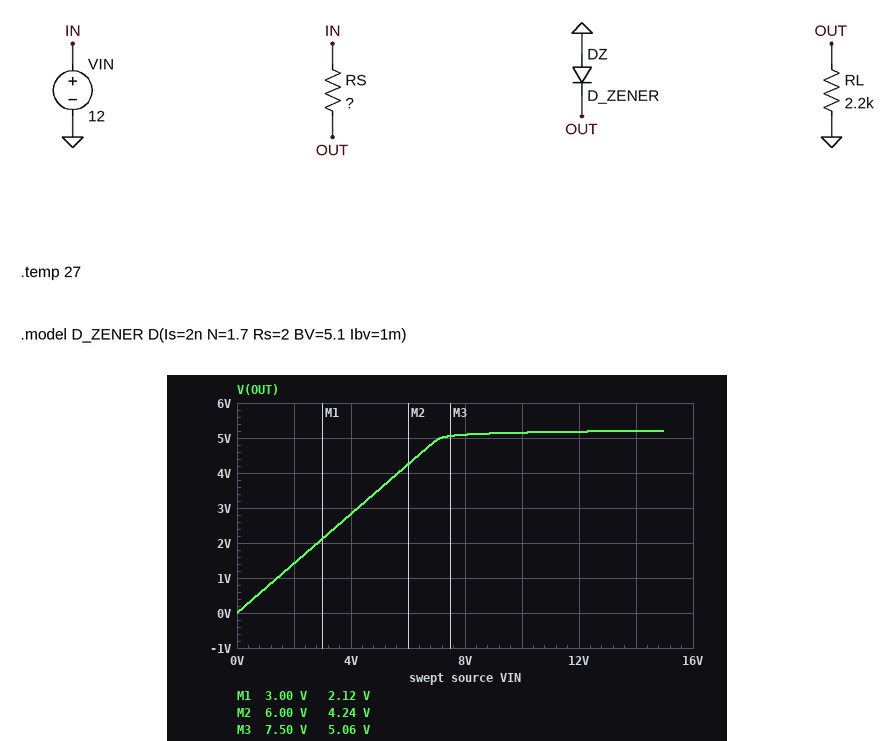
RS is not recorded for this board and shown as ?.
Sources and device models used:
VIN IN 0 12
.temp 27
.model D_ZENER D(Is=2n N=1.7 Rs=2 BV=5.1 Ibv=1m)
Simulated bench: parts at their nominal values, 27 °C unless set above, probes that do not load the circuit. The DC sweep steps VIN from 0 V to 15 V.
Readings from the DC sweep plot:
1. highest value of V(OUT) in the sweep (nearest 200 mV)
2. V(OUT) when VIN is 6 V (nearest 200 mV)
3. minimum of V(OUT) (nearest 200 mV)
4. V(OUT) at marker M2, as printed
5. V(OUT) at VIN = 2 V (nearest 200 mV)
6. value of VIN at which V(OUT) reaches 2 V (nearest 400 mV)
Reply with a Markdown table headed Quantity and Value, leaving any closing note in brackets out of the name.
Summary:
| Quantity | Value |
|---|---|
| highest value of V(OUT) in the sweep | 5.2 V |
| V(OUT) when VIN is 6 V | 4.2 V |
| minimum of V(OUT) | 0 V |
| V(OUT) at marker M2, as printed | 4.24 V |
| V(OUT) at VIN = 2 V | 1.4 V |
| value of VIN at which V(OUT) reaches 2 V | 2.8 V |
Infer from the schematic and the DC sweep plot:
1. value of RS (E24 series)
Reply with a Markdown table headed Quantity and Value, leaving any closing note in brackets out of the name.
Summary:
| Quantity | Value |
|---|---|
| value of RS | 910 Ω |
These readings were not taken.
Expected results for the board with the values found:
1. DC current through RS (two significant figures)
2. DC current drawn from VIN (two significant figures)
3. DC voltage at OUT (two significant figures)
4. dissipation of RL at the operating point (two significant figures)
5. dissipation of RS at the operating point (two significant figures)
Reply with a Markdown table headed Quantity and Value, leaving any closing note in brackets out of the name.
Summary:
| Quantity | Value |
|---|---|
| DC current through RS | 7.5 mA |
| DC current drawn from VIN | 7.5 mA |
| DC voltage at OUT | 5.2 V |
| dissipation of RL at the operating point | 12 mW |
| dissipation of RS at the operating point | 51 mW |
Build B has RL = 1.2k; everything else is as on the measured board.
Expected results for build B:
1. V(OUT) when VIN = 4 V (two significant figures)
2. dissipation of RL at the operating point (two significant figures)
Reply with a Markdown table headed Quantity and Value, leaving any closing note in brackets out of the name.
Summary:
| Quantity | Value |
|---|---|
| V(OUT) when VIN = 4 V | 2.3 V |
| dissipation of RL at the operating point | 22 mW |
